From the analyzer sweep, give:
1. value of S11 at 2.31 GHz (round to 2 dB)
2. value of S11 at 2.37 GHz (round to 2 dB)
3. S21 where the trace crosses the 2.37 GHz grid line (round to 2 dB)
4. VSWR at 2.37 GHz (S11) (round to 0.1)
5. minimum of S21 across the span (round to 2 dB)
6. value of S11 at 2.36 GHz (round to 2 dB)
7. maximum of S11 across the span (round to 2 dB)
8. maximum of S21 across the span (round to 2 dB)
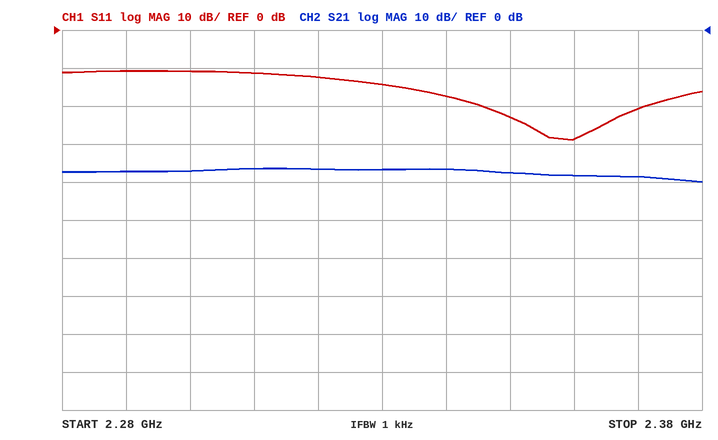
-12 dB
-20 dB
-38 dB
1.2
-40 dB
-28 dB
-10 dB
-36 dB
